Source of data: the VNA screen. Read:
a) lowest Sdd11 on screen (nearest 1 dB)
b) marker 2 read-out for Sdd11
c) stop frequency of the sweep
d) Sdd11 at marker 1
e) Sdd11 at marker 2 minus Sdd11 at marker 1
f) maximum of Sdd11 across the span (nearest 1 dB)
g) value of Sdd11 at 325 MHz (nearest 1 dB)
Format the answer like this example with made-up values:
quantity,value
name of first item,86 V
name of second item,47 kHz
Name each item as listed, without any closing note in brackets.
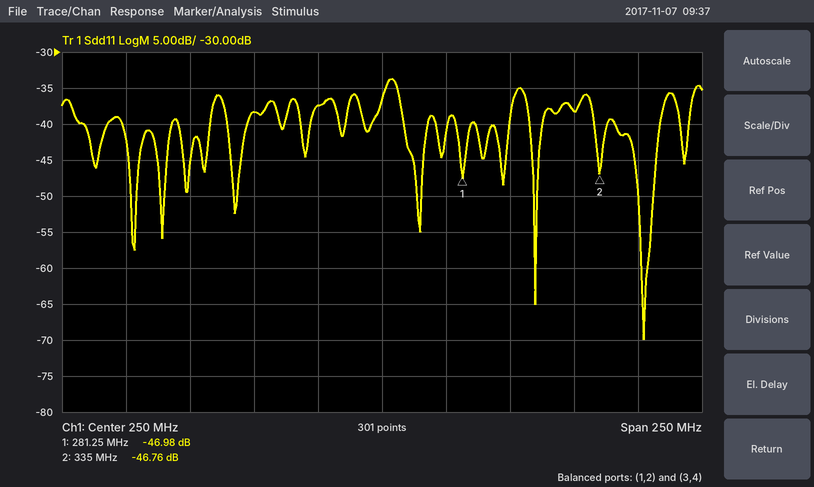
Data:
quantity,value
lowest Sdd11 on screen,-70 dB
marker 2 read-out for Sdd11,-46.76 dB
stop frequency of the sweep,375 MHz
Sdd11 at marker 1,-46.98 dB
Sdd11 at marker 2 minus Sdd11 at marker 1,0.22 dB
maximum of Sdd11 across the span,-34 dB
value of Sdd11 at 325 MHz,-38 dB
